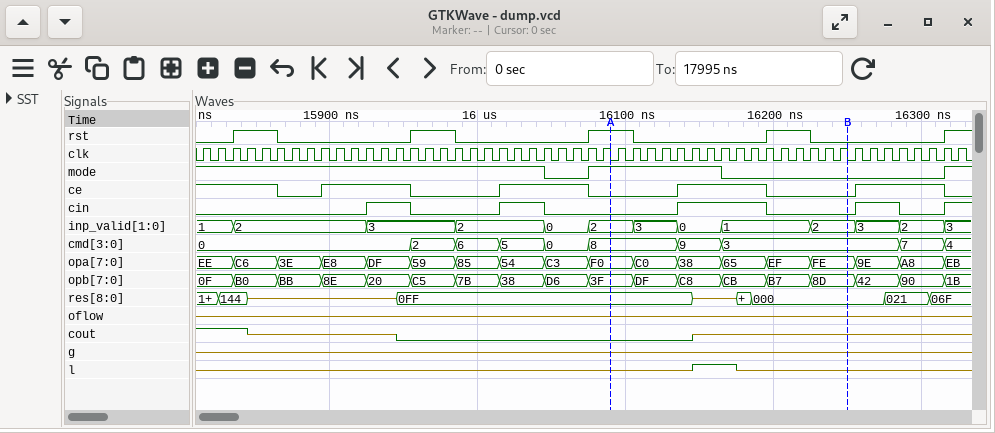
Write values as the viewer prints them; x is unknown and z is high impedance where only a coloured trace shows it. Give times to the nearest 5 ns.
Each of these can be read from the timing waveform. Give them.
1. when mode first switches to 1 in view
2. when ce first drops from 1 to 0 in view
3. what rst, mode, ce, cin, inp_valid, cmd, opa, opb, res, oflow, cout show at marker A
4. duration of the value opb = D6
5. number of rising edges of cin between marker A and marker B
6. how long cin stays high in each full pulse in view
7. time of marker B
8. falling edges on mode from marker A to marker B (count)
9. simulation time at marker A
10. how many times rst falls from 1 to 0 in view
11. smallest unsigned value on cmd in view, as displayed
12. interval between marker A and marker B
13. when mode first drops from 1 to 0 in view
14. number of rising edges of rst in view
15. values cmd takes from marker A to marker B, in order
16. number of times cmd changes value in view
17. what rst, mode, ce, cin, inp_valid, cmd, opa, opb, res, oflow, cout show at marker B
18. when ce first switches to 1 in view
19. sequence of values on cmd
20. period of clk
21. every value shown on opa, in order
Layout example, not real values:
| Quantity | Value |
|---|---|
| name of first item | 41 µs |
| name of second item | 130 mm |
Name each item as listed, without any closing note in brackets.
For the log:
| Quantity | Value |
|---|---|
| when mode first switches to 1 in view | 16075 ns |
| when ce first drops from 1 to 0 in view | 15865 ns |
| what rst, mode, ce, cin, inp_valid, cmd, opa, opb, res, oflow, cout show at marker A | rst=1, mode=1, ce=0, cin=0, inp_valid=2, cmd=8, opa=F0, opb=3F, res=0FF, oflow=z, cout=0 |
| duration of the value opb = D6 | 30 ns |
| number of rising edges of cin between marker A and marker B | 1 |
| how long cin stays high in each full pulse in view | 30 ns, 30 ns, 60 ns, 30 ns |
| time of marker B | 16250 ns |
| falling edges on mode from marker A to marker B | 1 |
| simulation time at marker A | 16090 ns |
| how many times rst falls from 1 to 0 in view | 4 |
| smallest unsigned value on cmd in view, as displayed | 0 |
| interval between marker A and marker B | 160 ns |
| when mode first drops from 1 to 0 in view | 16045 ns |
| number of rising edges of rst in view | 5 |
| values cmd takes from marker A to marker B, in order | 8, 9, 3 |
| number of times cmd changes value in view | 9 |
| what rst, mode, ce, cin, inp_valid, cmd, opa, opb, res, oflow, cout show at marker B | rst=0, mode=0, ce=0, cin=0, inp_valid=2, cmd=3, opa=FE, opb=8D, res=000, oflow=z, cout=z |
| when ce first switches to 1 in view | 15895 ns |
| sequence of values on cmd | 0, 2, 6, 5, 0, 8, 9, 3, 7, 4 |
| period of clk | 10 ns |
| every value shown on opa, in order | EE, C6, 3E, E8, DF, 59, 85, 54, C3, F0, C0, 38, 65, EF, FE, 9E, A8, EB |
